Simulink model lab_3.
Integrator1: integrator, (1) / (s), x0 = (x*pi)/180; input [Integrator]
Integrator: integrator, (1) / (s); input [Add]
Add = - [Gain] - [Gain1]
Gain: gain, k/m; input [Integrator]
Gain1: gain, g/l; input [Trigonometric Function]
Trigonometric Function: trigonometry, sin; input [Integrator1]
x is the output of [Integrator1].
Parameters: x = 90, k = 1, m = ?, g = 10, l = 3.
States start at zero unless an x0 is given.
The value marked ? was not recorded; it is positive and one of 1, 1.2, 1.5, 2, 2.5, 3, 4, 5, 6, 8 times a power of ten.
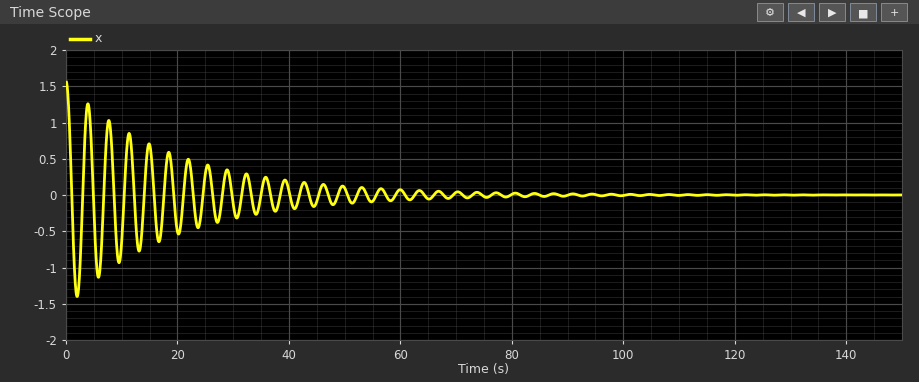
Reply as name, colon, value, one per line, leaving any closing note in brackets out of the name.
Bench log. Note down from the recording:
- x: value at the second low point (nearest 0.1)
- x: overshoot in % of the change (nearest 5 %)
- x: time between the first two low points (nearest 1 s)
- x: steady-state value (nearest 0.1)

x: value at the second low point: -1.1
x: overshoot in % of the change: 90 %
x: time between the first two low points: 4 s
x: steady-state value: 0.0
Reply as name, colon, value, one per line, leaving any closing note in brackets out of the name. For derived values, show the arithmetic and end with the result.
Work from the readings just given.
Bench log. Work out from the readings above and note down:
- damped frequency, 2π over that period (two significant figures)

damped frequency, 2π over that period: 2π / 4 = 1.6 rad/s
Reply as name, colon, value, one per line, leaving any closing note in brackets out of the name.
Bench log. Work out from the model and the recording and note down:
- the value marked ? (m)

the value marked ?: 10
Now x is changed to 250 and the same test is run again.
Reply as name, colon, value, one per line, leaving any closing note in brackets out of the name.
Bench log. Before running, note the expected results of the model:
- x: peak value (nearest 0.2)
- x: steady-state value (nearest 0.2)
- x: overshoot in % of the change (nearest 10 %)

x: peak value: 8.0
x: steady-state value: 6.2
x: overshoot in % of the change: 90 %
